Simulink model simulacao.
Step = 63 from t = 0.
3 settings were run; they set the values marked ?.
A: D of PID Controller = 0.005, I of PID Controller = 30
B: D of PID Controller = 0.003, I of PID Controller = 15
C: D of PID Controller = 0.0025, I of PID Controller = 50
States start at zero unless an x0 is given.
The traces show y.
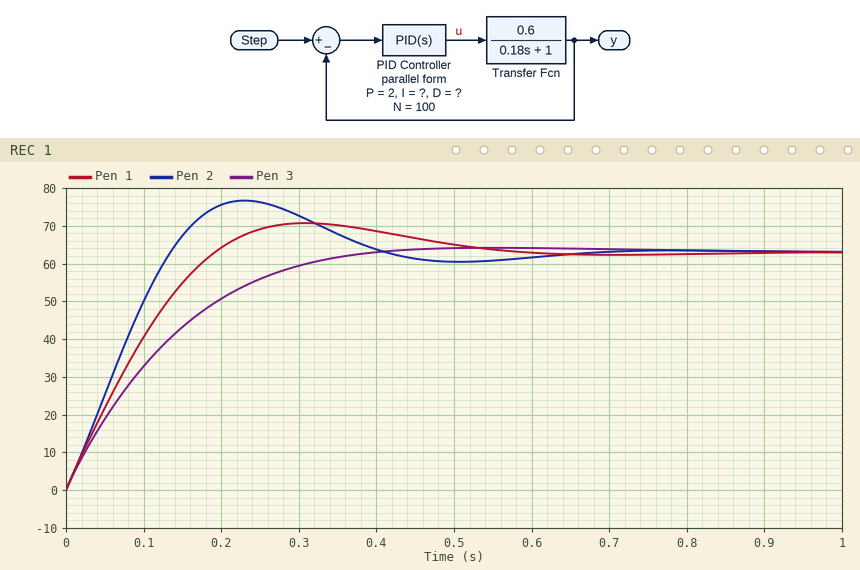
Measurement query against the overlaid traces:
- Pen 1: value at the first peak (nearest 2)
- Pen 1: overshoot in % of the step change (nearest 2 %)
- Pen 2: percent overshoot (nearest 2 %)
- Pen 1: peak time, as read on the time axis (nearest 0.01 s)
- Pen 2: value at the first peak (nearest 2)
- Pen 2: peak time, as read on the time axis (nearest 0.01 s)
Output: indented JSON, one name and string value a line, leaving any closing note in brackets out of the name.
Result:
{
  "Pen 1: value at the first peak": "70",
  "Pen 1: overshoot in % of the step change": "12 %",
  "Pen 2: percent overshoot": "22 %",
  "Pen 1: peak time, as read on the time axis": "0.31 s",
  "Pen 2: value at the first peak": "76",
  "Pen 2: peak time, as read on the time axis": "0.23 s"
}
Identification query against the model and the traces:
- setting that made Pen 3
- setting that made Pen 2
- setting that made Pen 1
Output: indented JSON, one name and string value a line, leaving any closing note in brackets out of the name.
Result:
{
  "setting that made Pen 3": "B",
  "setting that made Pen 2": "C",
  "setting that made Pen 1": "A"
}
